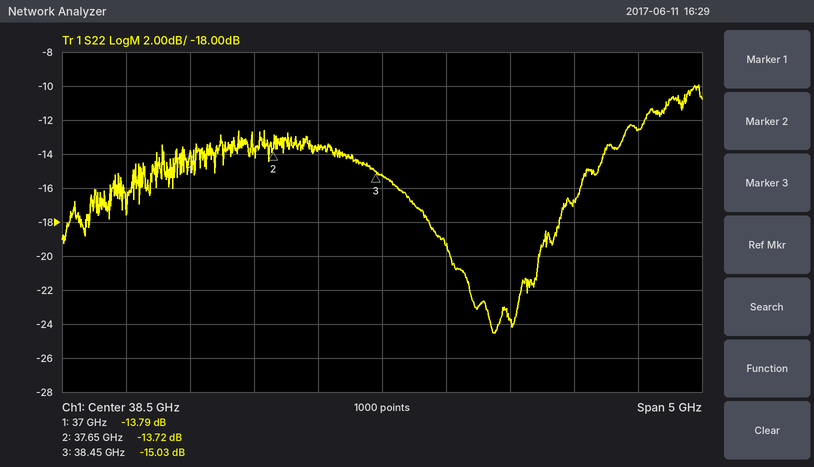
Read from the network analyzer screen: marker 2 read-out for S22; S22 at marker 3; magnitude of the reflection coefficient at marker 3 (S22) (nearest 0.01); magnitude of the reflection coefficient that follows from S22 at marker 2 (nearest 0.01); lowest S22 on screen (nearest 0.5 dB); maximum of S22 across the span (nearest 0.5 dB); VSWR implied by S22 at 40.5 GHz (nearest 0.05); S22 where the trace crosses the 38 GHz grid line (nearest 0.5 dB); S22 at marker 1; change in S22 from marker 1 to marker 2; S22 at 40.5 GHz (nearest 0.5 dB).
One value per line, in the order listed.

-13.72 dB
-15.03 dB
0.18
0.21
-24.5 dB
-10.0 dB
1.60
-13.5 dB
-13.79 dB
0.07 dB
-12.5 dB
